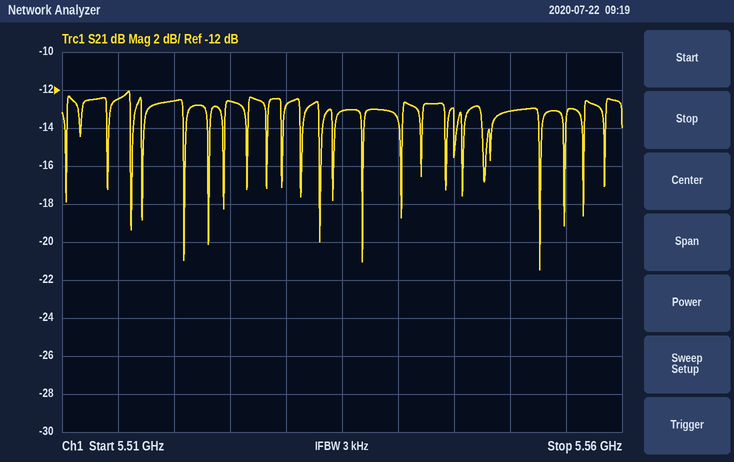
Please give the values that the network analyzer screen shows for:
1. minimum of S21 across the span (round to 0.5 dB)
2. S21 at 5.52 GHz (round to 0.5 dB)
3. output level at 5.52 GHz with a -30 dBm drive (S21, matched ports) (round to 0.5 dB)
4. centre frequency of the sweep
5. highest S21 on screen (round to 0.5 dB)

-21.5 dB
-12.5 dB
-42.5 dBm
5.535 GHz
-12.0 dB
